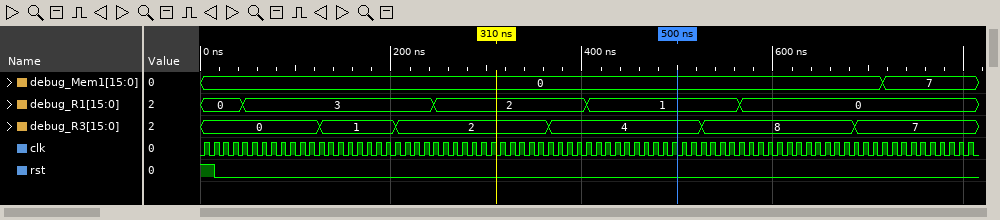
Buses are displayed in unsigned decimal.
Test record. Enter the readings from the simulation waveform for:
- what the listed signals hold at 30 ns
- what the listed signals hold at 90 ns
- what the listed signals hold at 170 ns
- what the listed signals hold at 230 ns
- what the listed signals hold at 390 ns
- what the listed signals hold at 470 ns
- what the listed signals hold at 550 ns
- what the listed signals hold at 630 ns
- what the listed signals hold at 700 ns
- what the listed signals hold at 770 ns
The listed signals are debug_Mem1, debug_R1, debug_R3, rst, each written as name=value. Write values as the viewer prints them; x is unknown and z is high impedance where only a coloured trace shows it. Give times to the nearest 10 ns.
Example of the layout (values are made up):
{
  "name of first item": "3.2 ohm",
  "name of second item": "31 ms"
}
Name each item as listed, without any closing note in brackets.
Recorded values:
{
  "what the listed signals hold at 30 ns": "debug_Mem1=0, debug_R1=0, debug_R3=0, rst=0",
  "what the listed signals hold at 90 ns": "debug_Mem1=0, debug_R1=3, debug_R3=0, rst=0",
  "what the listed signals hold at 170 ns": "debug_Mem1=0, debug_R1=3, debug_R3=1, rst=0",
  "what the listed signals hold at 230 ns": "debug_Mem1=0, debug_R1=3, debug_R3=2, rst=0",
  "what the listed signals hold at 390 ns": "debug_Mem1=0, debug_R1=2, debug_R3=4, rst=0",
  "what the listed signals hold at 470 ns": "debug_Mem1=0, debug_R1=1, debug_R3=4, rst=0",
  "what the listed signals hold at 550 ns": "debug_Mem1=0, debug_R1=1, debug_R3=8, rst=0",
  "what the listed signals hold at 630 ns": "debug_Mem1=0, debug_R1=0, debug_R3=8, rst=0",
  "what the listed signals hold at 700 ns": "debug_Mem1=0, debug_R1=0, debug_R3=7, rst=0",
  "what the listed signals hold at 770 ns": "debug_Mem1=7, debug_R1=0, debug_R3=7, rst=0"
}
